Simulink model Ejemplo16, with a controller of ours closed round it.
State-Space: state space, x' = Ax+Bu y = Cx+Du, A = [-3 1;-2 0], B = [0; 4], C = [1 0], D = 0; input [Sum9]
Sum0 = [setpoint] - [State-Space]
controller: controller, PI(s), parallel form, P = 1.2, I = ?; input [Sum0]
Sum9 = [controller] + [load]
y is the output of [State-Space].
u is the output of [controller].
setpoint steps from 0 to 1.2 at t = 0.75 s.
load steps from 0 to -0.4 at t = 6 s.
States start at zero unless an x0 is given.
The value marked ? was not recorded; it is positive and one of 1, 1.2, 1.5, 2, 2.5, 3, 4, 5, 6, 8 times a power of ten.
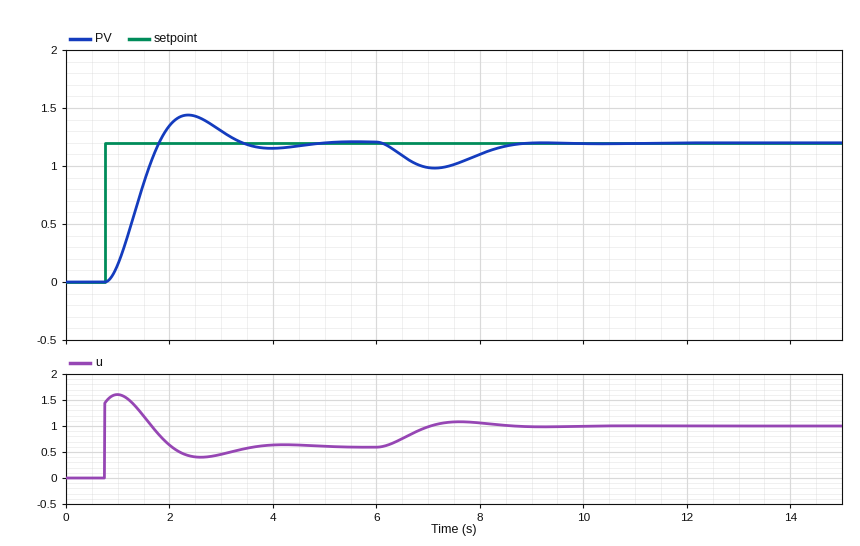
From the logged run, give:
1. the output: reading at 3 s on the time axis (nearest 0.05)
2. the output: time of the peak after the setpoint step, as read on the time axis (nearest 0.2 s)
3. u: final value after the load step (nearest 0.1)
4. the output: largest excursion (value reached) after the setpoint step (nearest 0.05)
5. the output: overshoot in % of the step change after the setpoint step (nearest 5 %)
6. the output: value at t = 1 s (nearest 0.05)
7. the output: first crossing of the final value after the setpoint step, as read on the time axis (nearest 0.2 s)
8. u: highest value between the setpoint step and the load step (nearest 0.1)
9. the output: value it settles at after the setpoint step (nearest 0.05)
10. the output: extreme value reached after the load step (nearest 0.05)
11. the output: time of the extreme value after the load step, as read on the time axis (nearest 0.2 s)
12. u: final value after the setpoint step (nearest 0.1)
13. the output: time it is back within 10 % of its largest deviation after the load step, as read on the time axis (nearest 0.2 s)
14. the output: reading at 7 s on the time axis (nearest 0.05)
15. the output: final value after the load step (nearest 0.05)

1.30
2.4 s
1.0
1.45
20 %
0.15
1.8 s
1.6
1.20
1.00
7.2 s
0.6
8.6 s
1.00
1.20
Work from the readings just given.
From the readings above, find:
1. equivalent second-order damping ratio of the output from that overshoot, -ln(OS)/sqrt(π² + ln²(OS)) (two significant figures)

0.46
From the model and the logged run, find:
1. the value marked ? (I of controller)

1.2
